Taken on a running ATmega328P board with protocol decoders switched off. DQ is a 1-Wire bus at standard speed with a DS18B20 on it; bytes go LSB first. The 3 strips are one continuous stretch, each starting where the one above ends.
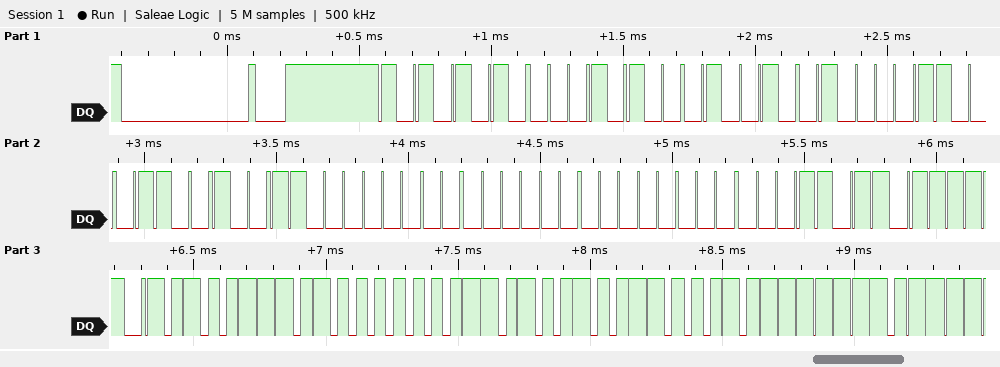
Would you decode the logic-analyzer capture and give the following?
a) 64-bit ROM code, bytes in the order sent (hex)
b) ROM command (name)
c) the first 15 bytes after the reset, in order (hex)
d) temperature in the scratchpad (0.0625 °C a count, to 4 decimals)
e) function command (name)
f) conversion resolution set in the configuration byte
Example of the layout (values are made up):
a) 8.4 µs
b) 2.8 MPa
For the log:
a) 28 92 30 26 03 00 00 D8
b) Match ROM
c) 55 28 92 30 26 03 00 00 D8 BE 72 01 4B 46 7F
d) 23.1250 °C
e) Read Scratchpad
f) 12 bits
